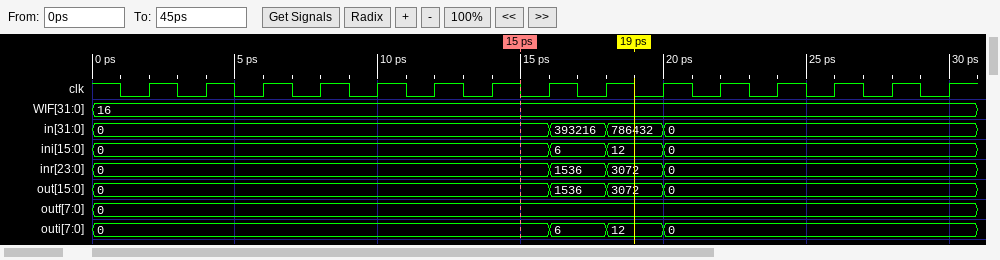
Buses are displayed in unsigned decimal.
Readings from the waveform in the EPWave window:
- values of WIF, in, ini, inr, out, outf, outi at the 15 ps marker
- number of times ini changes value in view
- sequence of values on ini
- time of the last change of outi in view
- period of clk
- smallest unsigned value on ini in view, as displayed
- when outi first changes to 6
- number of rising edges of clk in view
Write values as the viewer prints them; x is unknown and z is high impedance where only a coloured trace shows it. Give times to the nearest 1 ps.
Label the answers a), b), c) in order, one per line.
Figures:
a) WIF=16, in=0, ini=0, inr=0, out=0, outf=0, outi=0
b) 3
c) 0, 6, 12, 0
d) 20 ps
e) 2 ps
f) 0
g) 16 ps
h) 15
